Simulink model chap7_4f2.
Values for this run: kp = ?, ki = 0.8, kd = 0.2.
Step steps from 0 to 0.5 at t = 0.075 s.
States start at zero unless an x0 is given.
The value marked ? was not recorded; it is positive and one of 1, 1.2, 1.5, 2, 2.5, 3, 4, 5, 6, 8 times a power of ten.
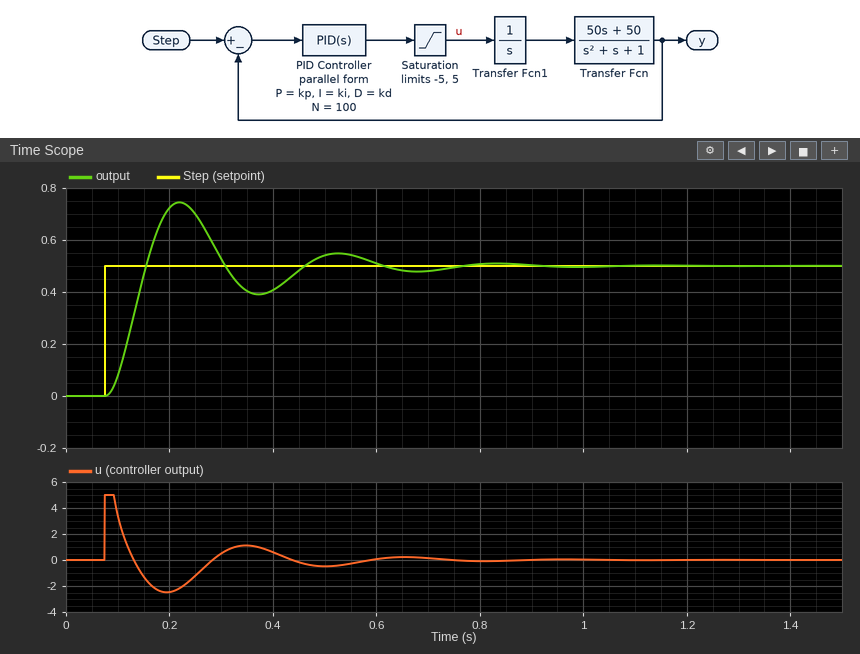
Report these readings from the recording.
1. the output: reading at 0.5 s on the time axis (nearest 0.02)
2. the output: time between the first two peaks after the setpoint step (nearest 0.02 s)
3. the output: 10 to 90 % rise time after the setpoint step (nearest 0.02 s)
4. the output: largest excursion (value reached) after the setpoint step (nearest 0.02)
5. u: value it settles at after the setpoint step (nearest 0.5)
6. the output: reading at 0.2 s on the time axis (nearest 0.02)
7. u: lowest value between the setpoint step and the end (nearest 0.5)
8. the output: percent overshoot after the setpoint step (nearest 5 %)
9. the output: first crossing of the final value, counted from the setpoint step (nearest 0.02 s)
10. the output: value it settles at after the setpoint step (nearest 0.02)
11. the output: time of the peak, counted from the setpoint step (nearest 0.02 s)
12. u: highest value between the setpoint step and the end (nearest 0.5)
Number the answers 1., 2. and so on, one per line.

1. 0.54
2. 0.30 s
3. 0.06 s
4. 0.74
5. 0.0
6. 0.72
7. -2.5
8. 50 %
9. 0.08 s
10. 0.50
11. 0.14 s
12. 5.0
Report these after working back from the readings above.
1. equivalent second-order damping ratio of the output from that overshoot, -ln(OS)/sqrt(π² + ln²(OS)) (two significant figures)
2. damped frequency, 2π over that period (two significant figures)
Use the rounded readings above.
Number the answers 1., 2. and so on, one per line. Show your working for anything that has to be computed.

1. ln(0.5) = -0.693; 0.693 / sqrt(9.870 + 0.480) = 0.22
2. 2π / 0.3 = 21 rad/s
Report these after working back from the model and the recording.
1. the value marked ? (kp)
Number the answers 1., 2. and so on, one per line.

1. 8
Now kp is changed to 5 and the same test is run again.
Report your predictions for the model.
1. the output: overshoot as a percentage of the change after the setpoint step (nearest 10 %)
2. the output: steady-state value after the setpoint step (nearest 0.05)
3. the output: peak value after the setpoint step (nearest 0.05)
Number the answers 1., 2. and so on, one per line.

1. 40 %
2. 0.50
3. 0.70
